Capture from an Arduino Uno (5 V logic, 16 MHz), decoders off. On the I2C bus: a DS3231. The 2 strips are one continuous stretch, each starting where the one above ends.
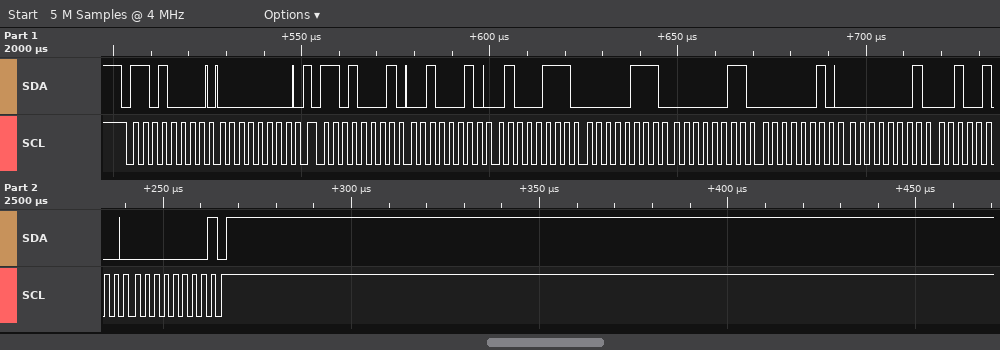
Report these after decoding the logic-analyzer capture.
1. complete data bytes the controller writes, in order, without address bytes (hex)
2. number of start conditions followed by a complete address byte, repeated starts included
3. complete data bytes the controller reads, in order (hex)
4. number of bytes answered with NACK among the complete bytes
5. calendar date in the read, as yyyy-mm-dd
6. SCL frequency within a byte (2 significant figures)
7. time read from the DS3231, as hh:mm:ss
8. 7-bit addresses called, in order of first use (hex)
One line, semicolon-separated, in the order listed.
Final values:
00; 2; 22 47 07 03 02 01 24 00; 1; 2024-01-02; 400 kHz; 07:47:22; 0x68
